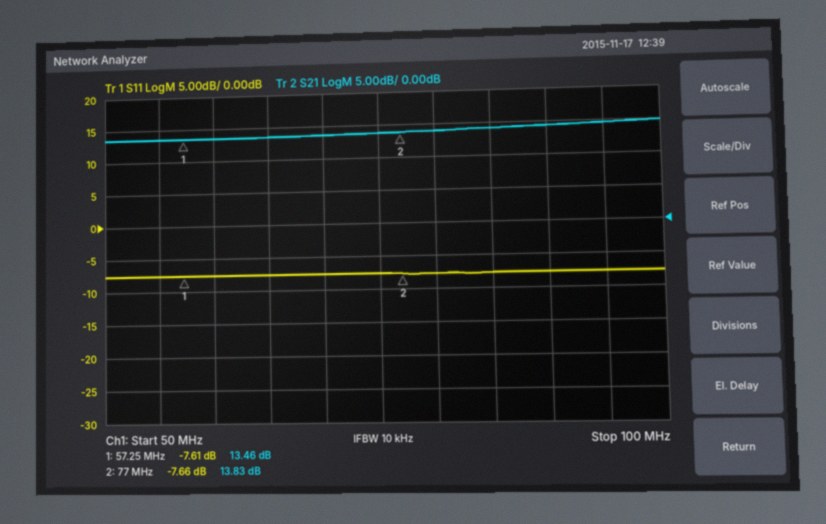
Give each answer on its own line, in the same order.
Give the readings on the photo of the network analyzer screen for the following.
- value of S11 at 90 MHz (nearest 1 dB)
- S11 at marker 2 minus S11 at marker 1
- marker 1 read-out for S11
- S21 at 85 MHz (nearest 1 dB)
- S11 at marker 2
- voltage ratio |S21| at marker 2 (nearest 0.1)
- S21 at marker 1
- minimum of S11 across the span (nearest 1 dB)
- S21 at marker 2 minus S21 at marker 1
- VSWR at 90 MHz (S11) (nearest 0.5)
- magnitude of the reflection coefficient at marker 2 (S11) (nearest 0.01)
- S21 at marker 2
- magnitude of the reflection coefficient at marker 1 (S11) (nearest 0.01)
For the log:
-8 dB
-0.05 dB
-7.61 dB
14 dB
-7.66 dB
4.9
13.46 dB
-8 dB
0.37 dB
2.5
0.41
13.83 dB
0.42
